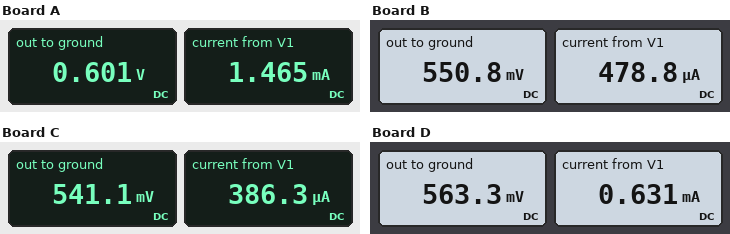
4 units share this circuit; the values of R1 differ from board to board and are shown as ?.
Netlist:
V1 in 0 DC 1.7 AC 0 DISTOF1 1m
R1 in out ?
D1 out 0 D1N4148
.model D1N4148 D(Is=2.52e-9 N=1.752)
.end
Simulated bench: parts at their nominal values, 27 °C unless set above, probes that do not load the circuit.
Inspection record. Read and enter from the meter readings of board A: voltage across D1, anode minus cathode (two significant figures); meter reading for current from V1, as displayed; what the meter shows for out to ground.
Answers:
600 mV
1.465 mA
0.601 V
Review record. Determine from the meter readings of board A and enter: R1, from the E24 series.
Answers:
750 Ω
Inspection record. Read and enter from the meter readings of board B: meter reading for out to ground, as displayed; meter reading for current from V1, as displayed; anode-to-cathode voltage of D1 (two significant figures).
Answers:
550.8 mV
478.8 µA
550 mV
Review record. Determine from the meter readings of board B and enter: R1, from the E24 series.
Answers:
2.4 kΩ
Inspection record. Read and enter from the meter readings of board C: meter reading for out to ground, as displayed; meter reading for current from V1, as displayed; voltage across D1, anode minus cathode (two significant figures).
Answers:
541.1 mV
386.3 µA
540 mV
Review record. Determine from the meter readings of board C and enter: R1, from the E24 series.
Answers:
3 kΩ
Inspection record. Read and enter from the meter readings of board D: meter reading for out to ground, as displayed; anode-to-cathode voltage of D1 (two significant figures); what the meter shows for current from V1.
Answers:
563.3 mV
560 mV
0.631 mA
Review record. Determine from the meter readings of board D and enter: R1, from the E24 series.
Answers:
1.8 kΩ
